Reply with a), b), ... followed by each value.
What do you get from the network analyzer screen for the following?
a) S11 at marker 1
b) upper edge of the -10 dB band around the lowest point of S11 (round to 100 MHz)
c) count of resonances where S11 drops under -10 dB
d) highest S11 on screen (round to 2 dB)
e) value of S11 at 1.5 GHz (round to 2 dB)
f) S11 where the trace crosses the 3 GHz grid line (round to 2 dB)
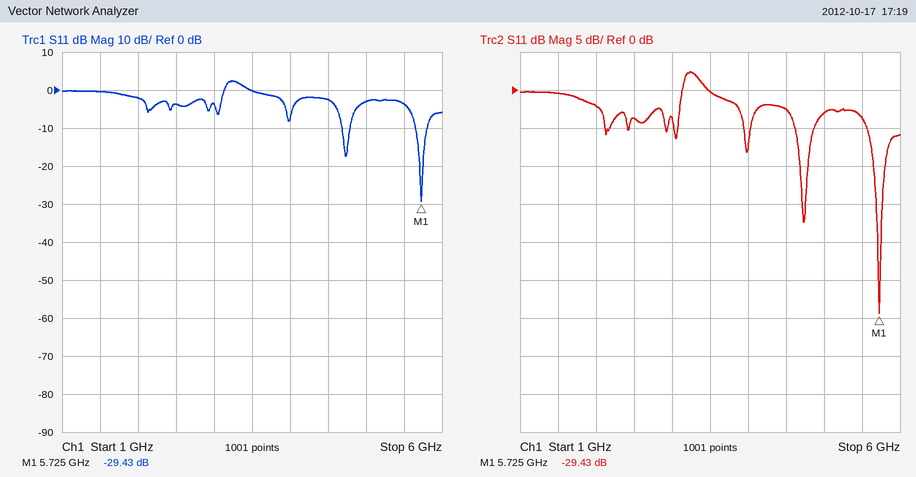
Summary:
a) -29.43 dB
b) 5.8 GHz
c) 2
d) 2 dB
e) 0 dB
f) -4 dB
